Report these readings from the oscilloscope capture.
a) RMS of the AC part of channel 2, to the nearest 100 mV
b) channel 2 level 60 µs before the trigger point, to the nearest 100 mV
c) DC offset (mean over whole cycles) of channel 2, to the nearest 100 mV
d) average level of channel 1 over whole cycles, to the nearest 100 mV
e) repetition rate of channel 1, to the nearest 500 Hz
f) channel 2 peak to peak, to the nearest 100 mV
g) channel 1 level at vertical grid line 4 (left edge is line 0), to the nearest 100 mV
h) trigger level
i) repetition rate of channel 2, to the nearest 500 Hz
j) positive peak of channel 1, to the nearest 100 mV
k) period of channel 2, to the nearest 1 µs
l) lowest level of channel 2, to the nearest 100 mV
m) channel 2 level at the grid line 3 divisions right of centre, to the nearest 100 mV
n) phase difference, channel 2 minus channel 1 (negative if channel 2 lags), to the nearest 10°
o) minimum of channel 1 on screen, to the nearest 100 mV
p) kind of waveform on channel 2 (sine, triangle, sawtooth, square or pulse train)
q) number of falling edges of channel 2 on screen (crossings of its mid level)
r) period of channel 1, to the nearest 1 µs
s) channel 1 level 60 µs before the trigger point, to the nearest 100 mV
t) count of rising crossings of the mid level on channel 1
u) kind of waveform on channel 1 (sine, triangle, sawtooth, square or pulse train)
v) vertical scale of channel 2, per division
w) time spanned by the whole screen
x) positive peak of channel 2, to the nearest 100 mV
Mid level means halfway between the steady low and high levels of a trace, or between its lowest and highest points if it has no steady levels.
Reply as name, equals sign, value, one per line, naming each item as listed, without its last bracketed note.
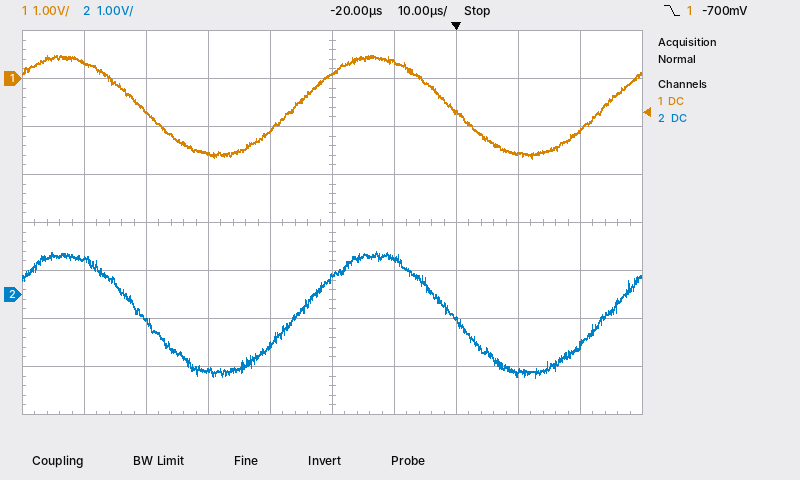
RMS of the AC part of channel 2, to the nearest 100 mV = 900 mV
channel 2 level 60 µs before the trigger point, to the nearest 100 mV = 700 mV
DC offset (mean over whole cycles) of channel 2, to the nearest 100 mV = -400 mV
average level of channel 1 over whole cycles, to the nearest 100 mV = -600 mV
repetition rate of channel 1, to the nearest 500 Hz = 20.0 kHz
channel 2 peak to peak, to the nearest 100 mV = 2.6 V
channel 1 level at vertical grid line 4 (left edge is line 0), to the nearest 100 mV = -1.1 V
trigger level = -700 mV
repetition rate of channel 2, to the nearest 500 Hz = 20.0 kHz
positive peak of channel 1, to the nearest 100 mV = 500 mV
period of channel 2, to the nearest 1 µs = 50 µs
lowest level of channel 2, to the nearest 100 mV = -1.7 V
channel 2 level at the grid line 3 divisions right of centre, to the nearest 100 mV = -1.6 V
phase difference, channel 2 minus channel 1 (negative if channel 2 lags), to the nearest 10° = 0°
minimum of channel 1 on screen, to the nearest 100 mV = -1.7 V
kind of waveform on channel 2 = sine
number of falling edges of channel 2 on screen = 2
period of channel 1, to the nearest 1 µs = 50 µs
channel 1 level 60 µs before the trigger point, to the nearest 100 mV = 300 mV
count of rising crossings of the mid level on channel 1 = 2
kind of waveform on channel 1 = sine
vertical scale of channel 2, per division = 1 V
time spanned by the whole screen = 100 µs
positive peak of channel 2, to the nearest 100 mV = 900 mV
